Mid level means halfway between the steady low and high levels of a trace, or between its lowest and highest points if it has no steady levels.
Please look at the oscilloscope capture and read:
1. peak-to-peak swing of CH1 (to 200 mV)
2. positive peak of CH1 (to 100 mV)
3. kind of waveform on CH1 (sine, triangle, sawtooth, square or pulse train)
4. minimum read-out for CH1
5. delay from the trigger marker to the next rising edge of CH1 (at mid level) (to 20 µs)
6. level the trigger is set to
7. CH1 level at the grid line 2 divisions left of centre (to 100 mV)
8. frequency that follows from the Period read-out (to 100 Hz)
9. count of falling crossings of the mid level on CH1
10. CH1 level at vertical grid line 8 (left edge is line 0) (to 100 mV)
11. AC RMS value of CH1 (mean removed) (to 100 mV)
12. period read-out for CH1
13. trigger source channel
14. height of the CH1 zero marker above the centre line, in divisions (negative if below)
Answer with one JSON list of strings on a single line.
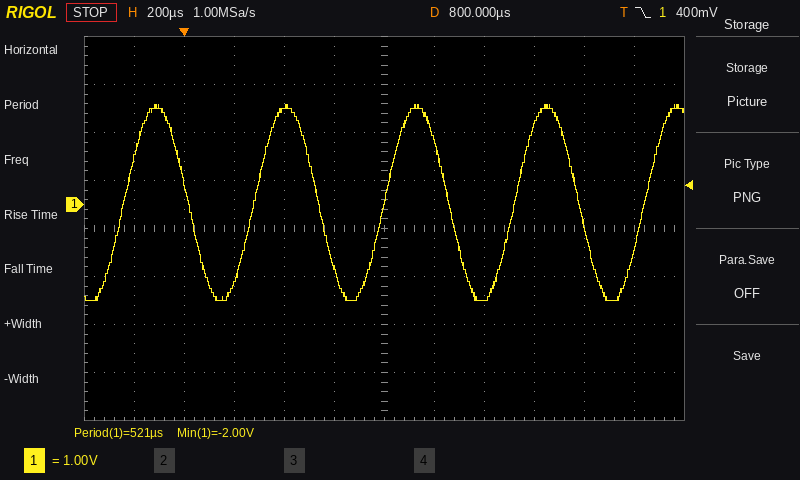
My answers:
["4.0 V", "2.1 V", "sine", "-2.00 V", "280 µs", "400 mV", "2.0 V", "1.9 kHz", "4", "-2.0 V", "1.4 V", "521 µs", "CH1", "+0.5 div"]
